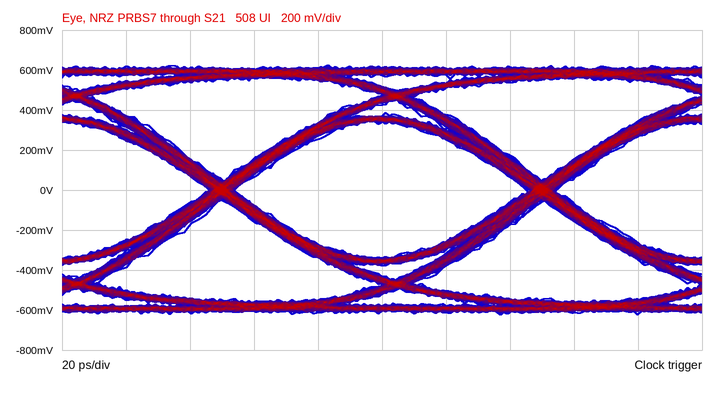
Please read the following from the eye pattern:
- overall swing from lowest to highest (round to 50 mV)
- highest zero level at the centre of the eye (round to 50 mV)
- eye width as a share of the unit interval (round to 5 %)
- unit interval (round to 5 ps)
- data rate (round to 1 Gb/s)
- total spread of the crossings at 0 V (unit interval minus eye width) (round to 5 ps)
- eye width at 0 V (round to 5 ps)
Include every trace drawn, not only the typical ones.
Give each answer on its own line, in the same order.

1.25 V
-350 mV
90 %
100 ps
10 Gb/s
10 ps
90 ps
